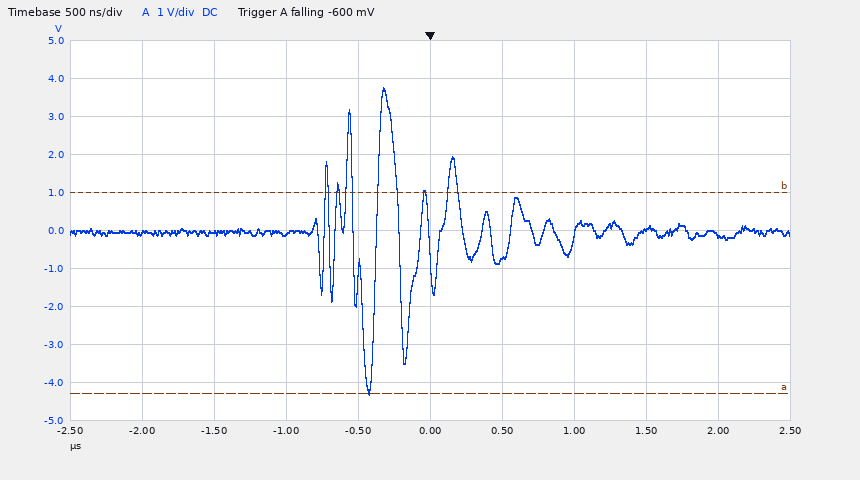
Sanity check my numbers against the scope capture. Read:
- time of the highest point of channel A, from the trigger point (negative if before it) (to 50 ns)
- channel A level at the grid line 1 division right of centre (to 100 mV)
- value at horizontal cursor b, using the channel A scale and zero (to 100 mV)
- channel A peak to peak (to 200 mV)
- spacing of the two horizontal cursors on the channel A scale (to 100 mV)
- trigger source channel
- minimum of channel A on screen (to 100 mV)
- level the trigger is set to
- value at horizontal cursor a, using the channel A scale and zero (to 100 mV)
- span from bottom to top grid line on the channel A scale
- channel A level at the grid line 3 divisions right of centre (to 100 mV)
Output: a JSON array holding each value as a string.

["-300 ns", "-800 mV", "1.0 V", "8.0 V", "5.3 V", "channel A", "-4.3 V", "-600 mV", "-4.3 V", "10 V", "0.0 V"]
